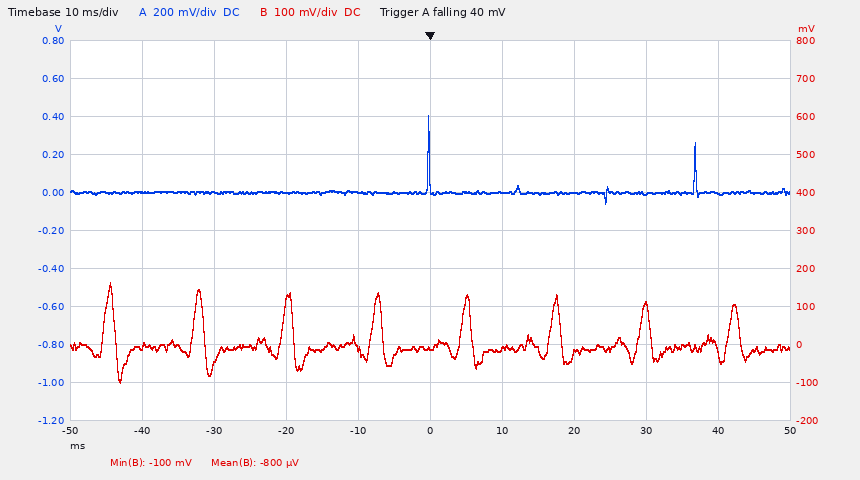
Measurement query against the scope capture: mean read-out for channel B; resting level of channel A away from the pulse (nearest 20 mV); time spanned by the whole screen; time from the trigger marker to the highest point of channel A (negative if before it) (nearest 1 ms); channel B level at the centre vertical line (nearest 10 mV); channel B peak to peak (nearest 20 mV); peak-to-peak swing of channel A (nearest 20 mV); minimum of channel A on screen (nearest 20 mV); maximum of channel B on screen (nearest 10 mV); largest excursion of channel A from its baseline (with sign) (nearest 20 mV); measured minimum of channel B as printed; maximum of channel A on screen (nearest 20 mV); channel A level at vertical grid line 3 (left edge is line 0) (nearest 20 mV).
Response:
-800 µV
0 mV
100 ms
0 ms
-10 mV
260 mV
460 mV
-60 mV
160 mV
+400 mV
-100 mV
400 mV
0 mV
